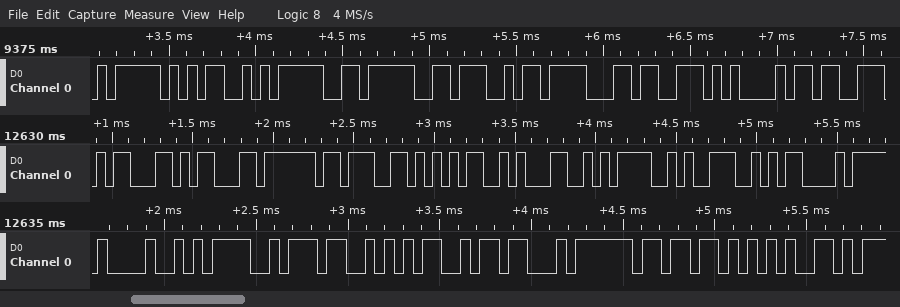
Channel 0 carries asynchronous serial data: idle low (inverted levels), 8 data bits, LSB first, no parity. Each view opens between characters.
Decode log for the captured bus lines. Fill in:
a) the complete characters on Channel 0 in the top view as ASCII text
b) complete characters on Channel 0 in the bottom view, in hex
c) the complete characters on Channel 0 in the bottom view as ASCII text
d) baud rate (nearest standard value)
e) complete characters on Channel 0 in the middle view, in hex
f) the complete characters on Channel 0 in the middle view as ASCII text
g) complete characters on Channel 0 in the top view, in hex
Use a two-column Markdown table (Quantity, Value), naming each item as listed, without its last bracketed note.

| Quantity | Value |
|---|---|
| the complete characters on Channel 0 in the top view as ASCII text | "AY00,8F/" |
| complete characters on Channel 0 in the bottom view, in hex | 6F, 61, 64, 65, 72, 20, 52, 4D |
| the complete characters on Channel 0 in the bottom view as ASCII text | "oader RM" |
| baud rate | 19200 baud |
| complete characters on Channel 0 in the middle view, in hex | 39, 39, 20, 4C, 65, 67, 61, 63, 79 |
| the complete characters on Channel 0 in the middle view as ASCII text | "99 Legacy" |
| complete characters on Channel 0 in the top view, in hex | 41, 59, 30, 30, 2C, 38, 46, 2F |
